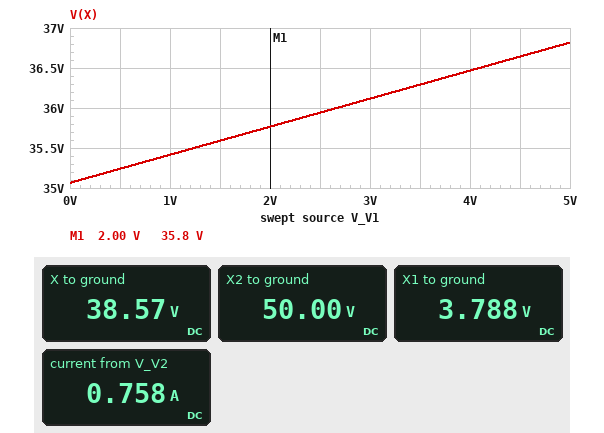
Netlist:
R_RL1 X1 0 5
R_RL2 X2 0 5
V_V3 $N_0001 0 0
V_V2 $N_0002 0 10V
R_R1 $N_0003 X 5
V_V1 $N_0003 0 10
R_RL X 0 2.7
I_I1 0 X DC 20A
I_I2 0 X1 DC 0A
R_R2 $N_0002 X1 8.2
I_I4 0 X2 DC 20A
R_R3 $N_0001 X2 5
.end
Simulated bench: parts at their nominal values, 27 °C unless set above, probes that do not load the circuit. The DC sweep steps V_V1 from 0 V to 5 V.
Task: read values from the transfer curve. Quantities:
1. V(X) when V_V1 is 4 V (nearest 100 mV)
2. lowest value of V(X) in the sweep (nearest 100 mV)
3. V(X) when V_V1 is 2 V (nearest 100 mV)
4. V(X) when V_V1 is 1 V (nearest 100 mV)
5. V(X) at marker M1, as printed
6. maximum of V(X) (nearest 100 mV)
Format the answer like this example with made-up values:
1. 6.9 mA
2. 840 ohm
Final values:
1. 36.5 V
2. 35.1 V
3. 35.8 V
4. 35.4 V
5. 35.8 V
6. 36.8 V
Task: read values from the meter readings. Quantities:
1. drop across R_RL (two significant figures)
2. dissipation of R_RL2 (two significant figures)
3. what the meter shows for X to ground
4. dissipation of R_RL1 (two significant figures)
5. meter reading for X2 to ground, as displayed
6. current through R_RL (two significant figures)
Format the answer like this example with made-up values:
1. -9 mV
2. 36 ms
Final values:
1. 39 V
2. 500 W
3. 38.57 V
4. 2.9 W
5. 50.00 V
6. 14 A
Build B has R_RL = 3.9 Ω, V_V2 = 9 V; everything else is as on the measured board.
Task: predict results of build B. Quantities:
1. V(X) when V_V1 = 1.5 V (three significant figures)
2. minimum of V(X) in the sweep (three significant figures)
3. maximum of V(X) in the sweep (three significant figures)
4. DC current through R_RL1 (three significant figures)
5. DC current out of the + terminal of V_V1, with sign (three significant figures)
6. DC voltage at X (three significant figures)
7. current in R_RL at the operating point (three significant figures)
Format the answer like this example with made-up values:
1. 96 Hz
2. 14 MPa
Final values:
1. 44.5 V
2. 43.8 V
3. 46.0 V
4. 682 mA
5. -7.64 A
6. 48.2 V
7. 12.4 A
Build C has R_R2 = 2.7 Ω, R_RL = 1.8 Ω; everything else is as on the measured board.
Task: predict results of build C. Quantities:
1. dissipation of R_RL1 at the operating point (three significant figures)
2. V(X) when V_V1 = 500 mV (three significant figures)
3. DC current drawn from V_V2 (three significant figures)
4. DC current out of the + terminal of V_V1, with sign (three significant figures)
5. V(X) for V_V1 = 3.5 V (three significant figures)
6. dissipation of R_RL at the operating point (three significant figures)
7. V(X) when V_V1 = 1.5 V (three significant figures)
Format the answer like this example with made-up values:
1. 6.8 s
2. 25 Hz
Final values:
1. 8.43 W
2. 26.6 V
3. 1.30 A
4. -3.82 A
5. 27.4 V
6. 471 W
7. 26.9 V
